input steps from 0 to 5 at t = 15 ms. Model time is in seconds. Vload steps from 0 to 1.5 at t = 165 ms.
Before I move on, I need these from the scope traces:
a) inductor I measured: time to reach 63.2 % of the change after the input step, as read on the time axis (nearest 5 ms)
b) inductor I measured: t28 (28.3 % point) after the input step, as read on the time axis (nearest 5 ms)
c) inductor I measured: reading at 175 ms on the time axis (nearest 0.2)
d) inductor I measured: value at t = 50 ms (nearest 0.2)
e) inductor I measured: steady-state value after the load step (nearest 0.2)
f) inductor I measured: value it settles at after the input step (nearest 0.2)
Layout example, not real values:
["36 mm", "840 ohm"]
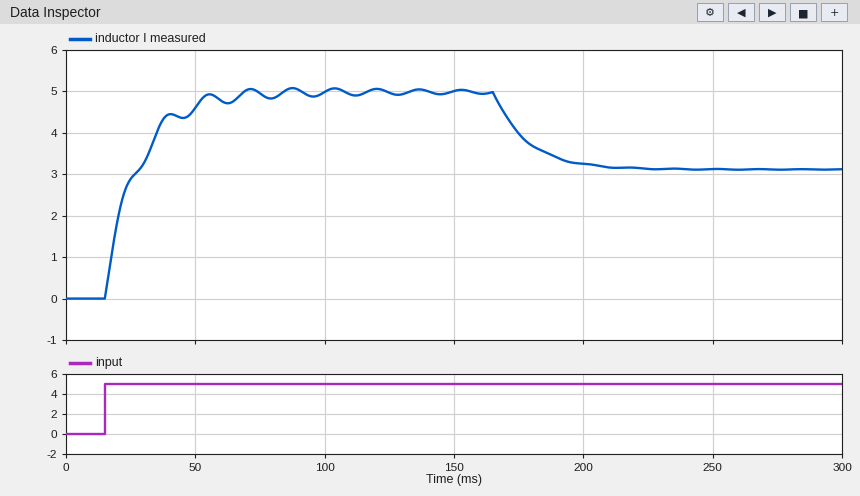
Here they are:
["30 ms", "20 ms", "4.0", "4.6", "3.2", "5.0"]
